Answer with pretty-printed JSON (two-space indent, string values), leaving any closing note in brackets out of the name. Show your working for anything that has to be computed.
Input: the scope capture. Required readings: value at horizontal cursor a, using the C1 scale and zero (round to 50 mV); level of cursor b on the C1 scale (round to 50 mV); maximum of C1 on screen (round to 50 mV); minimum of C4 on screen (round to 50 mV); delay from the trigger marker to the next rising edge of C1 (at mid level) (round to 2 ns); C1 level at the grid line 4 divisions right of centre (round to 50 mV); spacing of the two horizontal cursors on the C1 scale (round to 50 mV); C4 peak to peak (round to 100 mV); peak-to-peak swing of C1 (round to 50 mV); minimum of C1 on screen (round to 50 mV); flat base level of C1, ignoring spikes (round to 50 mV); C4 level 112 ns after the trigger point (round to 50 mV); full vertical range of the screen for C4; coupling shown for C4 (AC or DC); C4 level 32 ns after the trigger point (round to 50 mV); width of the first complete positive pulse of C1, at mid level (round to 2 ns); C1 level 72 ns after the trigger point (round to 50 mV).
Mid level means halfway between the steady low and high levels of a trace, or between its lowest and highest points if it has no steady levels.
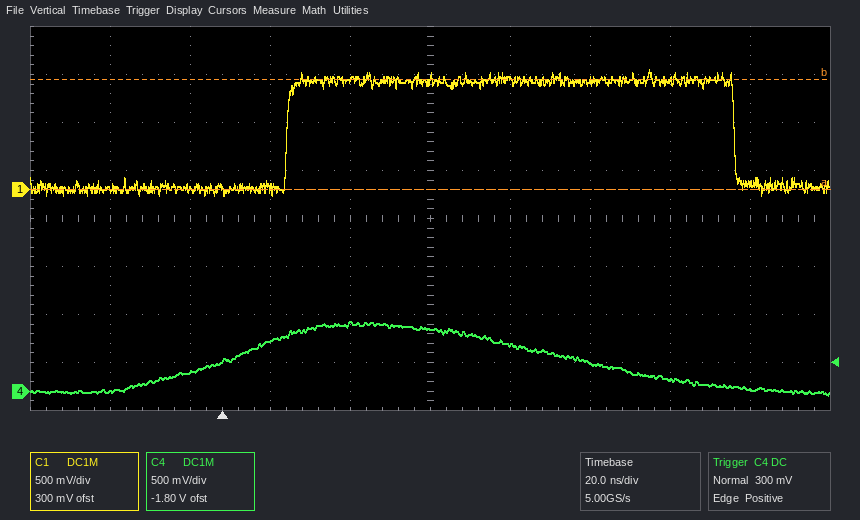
{
  "value at horizontal cursor a, using the C1 scale and zero": "0 mV",
  "level of cursor b on the C1 scale": "1.15 V",
  "maximum of C1 on screen": "1.25 V",
  "minimum of C4 on screen": "-50 mV",
  "delay from the trigger marker to the next rising edge of C1 (at mid level)": "16 ns",
  "C1 level at the grid line 4 divisions right of centre": "50 mV",
  "spacing of the two horizontal cursors on the C1 scale": "1.15 V",
  "C4 peak to peak": "800 mV",
  "peak-to-peak swing of C1": "1.25 V − (-50 mV) = 1.30 V",
  "minimum of C1 on screen": "-50 mV",
  "flat base level of C1, ignoring spikes": "0 mV",
  "C4 level 112 ns after the trigger point": "100 mV",
  "full vertical range of the screen for C4": "4 V",
  "coupling shown for C4": "DC",
  "C4 level 32 ns after the trigger point": "700 mV",
  "width of the first complete positive pulse of C1, at mid level": "112 ns",
  "C1 level 72 ns after the trigger point": "1.15 V"
}
